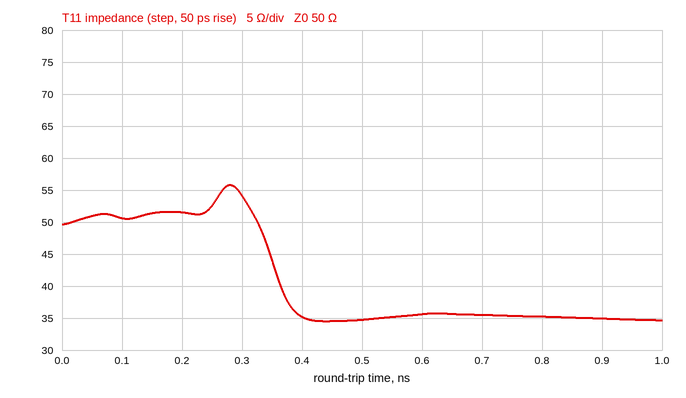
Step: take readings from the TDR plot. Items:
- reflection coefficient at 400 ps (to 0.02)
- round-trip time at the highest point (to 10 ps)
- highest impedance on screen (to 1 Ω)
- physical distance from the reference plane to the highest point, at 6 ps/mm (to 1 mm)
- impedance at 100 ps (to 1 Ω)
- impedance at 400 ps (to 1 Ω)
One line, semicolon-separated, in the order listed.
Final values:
-0.18; 280 ps; 56 Ω; 23 mm; 51 Ω; 35 Ω
